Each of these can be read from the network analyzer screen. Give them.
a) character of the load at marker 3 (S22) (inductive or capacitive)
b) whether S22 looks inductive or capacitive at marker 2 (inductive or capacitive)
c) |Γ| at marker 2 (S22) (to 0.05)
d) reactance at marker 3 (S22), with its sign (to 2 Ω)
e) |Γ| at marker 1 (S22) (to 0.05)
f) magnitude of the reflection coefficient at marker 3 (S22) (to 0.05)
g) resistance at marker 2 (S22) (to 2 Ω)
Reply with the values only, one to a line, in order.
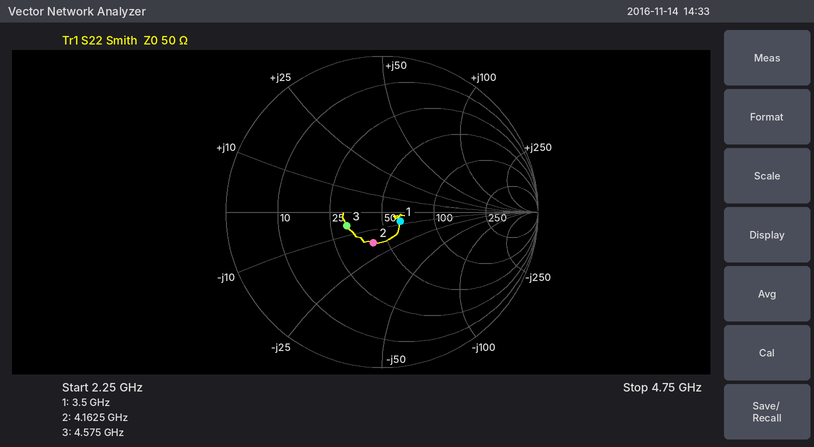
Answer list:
capacitive
capacitive
0.20
-6 Ω
0.15
0.25
42 Ω
